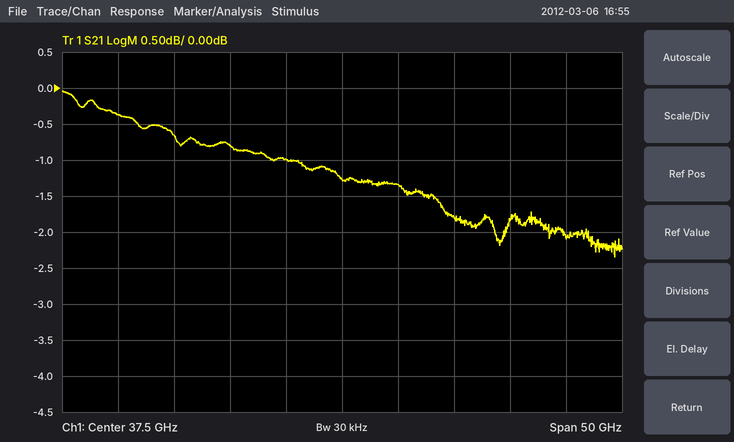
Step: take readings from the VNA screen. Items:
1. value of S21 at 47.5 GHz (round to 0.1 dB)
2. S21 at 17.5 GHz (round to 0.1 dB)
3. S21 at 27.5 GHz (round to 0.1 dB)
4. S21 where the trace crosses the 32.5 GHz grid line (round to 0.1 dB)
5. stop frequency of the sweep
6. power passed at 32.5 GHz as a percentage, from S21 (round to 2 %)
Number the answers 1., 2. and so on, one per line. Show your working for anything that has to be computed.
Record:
1. -1.8 dB
2. -0.4 dB
3. -0.8 dB
4. -1.0 dB
5. 62.5 GHz
6. 10^(-1/10) ≈ 79.4 %, so 80 % to the nearest 2 %
